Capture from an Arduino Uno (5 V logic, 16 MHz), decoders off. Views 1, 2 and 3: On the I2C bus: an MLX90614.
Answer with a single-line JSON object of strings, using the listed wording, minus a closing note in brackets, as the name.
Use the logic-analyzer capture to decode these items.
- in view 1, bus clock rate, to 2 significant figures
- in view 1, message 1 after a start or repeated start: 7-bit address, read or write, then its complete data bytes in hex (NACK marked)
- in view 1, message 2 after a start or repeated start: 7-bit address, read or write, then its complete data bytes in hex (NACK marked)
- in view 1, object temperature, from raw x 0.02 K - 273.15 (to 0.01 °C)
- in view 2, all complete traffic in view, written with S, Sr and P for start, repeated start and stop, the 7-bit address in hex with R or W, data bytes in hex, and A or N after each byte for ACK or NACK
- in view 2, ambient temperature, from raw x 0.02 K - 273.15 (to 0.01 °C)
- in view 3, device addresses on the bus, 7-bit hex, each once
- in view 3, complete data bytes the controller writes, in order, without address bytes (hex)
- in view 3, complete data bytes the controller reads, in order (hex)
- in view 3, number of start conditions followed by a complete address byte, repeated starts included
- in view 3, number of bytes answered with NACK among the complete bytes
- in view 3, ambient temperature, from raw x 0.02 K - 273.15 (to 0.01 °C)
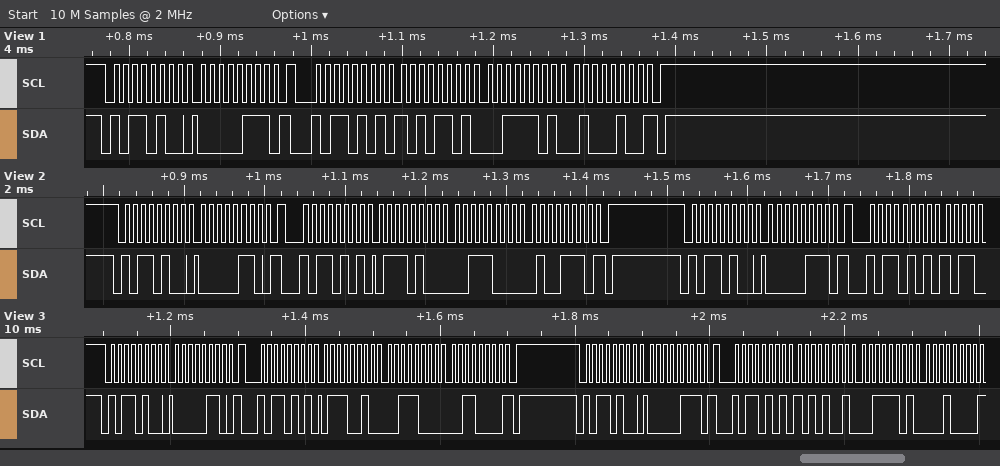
{"in view 1, bus clock rate, to 2 significant figures": "100 kHz", "in view 1, message 1 after a start or repeated start: 7-bit address, read or write, then its complete data bytes in hex": "0x5A write: 07", "in view 1, message 2 after a start or repeated start: 7-bit address, read or write, then its complete data bytes in hex": "0x5A read: AD 3D 44 NACK", "in view 1, object temperature, from raw x 0.02 K - 273.15": "42.63 °C", "in view 2, all complete traffic in view, written with S, Sr and P for start, repeated start and stop, the 7-bit address in hex with R or W, data bytes in hex, and A or N after each byte for ACK or NACK": "S 5AW A 06 A Sr 5AR A 74 A 38 A 4E N P S 5AW A 07 A Sr 5AR A", "in view 2, ambient temperature, from raw x 0.02 K - 273.15": "15.89 °C", "in view 3, device addresses on the bus, 7-bit hex, each once": "0x5A", "in view 3, complete data bytes the controller writes, in order, without address bytes": "06 07", "in view 3, complete data bytes the controller reads, in order": "72 38 30 A9 3D 10", "in view 3, number of start conditions followed by a complete address byte, repeated starts included": "4", "in view 3, number of bytes answered with NACK among the complete bytes": "2", "in view 3, ambient temperature, from raw x 0.02 K - 273.15": "15.85 °C"}
